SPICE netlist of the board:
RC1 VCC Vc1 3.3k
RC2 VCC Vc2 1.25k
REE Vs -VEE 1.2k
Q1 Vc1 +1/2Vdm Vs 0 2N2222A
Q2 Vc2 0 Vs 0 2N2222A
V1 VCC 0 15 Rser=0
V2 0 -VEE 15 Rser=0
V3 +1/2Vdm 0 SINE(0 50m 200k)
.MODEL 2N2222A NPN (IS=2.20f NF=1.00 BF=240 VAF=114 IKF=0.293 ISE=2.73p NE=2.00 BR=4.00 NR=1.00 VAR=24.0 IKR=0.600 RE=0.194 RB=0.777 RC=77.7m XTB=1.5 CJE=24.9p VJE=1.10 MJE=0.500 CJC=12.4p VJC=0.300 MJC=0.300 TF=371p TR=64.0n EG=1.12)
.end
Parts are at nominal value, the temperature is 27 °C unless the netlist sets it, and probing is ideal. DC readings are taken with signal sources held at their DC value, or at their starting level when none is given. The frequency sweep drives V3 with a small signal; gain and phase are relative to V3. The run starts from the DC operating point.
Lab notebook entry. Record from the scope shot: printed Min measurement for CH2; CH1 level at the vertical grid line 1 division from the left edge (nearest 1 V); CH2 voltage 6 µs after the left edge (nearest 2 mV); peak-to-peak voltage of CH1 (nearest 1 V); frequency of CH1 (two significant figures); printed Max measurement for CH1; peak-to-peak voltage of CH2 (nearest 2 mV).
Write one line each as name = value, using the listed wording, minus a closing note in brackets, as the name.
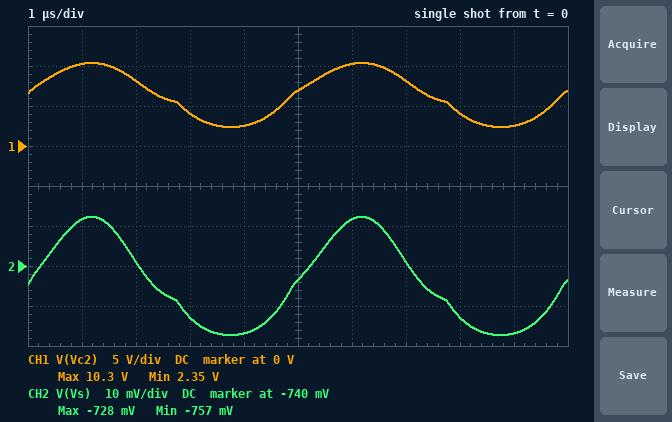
printed Min measurement for CH2 = -757 mV
CH1 level at the vertical grid line 1 division from the left edge = 10 V
CH2 voltage 6 µs after the left edge = -728 mV
peak-to-peak voltage of CH1 = 8 V
frequency of CH1 = 200 kHz
printed Max measurement for CH1 = 10.3 V
peak-to-peak voltage of CH2 = 30 mV
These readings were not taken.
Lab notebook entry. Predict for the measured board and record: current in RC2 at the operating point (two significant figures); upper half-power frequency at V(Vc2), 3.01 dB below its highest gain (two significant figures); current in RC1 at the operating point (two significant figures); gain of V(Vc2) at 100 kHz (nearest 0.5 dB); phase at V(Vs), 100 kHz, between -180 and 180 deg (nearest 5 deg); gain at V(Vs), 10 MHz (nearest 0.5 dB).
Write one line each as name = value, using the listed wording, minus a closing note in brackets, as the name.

current in RC2 at the operating point = 6.7 mA
upper half-power frequency at V(Vc2), 3.01 dB below its highest gain = 28 MHz
current in RC1 at the operating point = 4.8 mA
gain of V(Vc2) at 100 kHz = 34.0 dB
phase at V(Vs), 100 kHz, between -180 and 180 deg = 5 deg
gain at V(Vs), 10 MHz = -6.5 dB
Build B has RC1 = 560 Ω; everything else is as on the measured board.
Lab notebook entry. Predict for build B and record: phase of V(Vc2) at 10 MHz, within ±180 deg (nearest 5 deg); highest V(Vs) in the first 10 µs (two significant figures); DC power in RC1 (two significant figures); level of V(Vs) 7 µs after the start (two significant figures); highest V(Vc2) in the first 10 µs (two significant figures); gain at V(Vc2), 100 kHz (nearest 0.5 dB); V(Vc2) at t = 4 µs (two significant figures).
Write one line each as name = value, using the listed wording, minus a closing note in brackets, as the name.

phase of V(Vc2) at 10 MHz, within ±180 deg = -20 deg
highest V(Vs) in the first 10 µs = -710 mV
DC power in RC1 = 20 mW
level of V(Vs) 7 µs after the start = -720 mV
highest V(Vc2) in the first 10 µs = 13 V
gain at V(Vc2), 100 kHz = 42.0 dB
V(Vc2) at t = 4 µs = 2.6 V
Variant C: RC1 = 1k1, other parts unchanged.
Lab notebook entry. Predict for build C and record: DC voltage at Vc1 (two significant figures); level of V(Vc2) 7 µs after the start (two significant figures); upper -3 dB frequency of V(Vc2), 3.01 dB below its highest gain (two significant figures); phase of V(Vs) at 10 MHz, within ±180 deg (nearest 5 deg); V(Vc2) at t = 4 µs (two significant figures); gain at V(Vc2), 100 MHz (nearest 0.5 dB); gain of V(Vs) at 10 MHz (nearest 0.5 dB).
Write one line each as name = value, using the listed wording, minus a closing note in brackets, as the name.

DC voltage at Vc1 = 8.5 V
level of V(Vc2) 7 µs after the start = 11 V
upper -3 dB frequency of V(Vc2), 3.01 dB below its highest gain = 25 MHz
phase of V(Vs) at 10 MHz, within ±180 deg = 0 deg
V(Vc2) at t = 4 µs = 2.6 V
gain at V(Vc2), 100 MHz = 29.5 dB
gain of V(Vs) at 10 MHz = -6.0 dB
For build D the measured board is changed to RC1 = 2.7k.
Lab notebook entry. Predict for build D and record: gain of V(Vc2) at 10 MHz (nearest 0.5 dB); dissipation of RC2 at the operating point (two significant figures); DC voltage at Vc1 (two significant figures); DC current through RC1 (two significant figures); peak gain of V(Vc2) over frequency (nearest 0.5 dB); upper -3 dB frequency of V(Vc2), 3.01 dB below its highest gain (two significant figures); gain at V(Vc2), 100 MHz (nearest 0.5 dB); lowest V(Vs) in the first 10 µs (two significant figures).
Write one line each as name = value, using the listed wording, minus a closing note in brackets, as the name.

gain of V(Vc2) at 10 MHz = 41.0 dB
dissipation of RC2 at the operating point = 47 mW
DC voltage at Vc1 = -440 mV
DC current through RC1 = 5.7 mA
peak gain of V(Vc2) over frequency = 41.5 dB
upper -3 dB frequency of V(Vc2), 3.01 dB below its highest gain = 25 MHz
gain at V(Vc2), 100 MHz = 29.5 dB
lowest V(Vs) in the first 10 µs = -760 mV
